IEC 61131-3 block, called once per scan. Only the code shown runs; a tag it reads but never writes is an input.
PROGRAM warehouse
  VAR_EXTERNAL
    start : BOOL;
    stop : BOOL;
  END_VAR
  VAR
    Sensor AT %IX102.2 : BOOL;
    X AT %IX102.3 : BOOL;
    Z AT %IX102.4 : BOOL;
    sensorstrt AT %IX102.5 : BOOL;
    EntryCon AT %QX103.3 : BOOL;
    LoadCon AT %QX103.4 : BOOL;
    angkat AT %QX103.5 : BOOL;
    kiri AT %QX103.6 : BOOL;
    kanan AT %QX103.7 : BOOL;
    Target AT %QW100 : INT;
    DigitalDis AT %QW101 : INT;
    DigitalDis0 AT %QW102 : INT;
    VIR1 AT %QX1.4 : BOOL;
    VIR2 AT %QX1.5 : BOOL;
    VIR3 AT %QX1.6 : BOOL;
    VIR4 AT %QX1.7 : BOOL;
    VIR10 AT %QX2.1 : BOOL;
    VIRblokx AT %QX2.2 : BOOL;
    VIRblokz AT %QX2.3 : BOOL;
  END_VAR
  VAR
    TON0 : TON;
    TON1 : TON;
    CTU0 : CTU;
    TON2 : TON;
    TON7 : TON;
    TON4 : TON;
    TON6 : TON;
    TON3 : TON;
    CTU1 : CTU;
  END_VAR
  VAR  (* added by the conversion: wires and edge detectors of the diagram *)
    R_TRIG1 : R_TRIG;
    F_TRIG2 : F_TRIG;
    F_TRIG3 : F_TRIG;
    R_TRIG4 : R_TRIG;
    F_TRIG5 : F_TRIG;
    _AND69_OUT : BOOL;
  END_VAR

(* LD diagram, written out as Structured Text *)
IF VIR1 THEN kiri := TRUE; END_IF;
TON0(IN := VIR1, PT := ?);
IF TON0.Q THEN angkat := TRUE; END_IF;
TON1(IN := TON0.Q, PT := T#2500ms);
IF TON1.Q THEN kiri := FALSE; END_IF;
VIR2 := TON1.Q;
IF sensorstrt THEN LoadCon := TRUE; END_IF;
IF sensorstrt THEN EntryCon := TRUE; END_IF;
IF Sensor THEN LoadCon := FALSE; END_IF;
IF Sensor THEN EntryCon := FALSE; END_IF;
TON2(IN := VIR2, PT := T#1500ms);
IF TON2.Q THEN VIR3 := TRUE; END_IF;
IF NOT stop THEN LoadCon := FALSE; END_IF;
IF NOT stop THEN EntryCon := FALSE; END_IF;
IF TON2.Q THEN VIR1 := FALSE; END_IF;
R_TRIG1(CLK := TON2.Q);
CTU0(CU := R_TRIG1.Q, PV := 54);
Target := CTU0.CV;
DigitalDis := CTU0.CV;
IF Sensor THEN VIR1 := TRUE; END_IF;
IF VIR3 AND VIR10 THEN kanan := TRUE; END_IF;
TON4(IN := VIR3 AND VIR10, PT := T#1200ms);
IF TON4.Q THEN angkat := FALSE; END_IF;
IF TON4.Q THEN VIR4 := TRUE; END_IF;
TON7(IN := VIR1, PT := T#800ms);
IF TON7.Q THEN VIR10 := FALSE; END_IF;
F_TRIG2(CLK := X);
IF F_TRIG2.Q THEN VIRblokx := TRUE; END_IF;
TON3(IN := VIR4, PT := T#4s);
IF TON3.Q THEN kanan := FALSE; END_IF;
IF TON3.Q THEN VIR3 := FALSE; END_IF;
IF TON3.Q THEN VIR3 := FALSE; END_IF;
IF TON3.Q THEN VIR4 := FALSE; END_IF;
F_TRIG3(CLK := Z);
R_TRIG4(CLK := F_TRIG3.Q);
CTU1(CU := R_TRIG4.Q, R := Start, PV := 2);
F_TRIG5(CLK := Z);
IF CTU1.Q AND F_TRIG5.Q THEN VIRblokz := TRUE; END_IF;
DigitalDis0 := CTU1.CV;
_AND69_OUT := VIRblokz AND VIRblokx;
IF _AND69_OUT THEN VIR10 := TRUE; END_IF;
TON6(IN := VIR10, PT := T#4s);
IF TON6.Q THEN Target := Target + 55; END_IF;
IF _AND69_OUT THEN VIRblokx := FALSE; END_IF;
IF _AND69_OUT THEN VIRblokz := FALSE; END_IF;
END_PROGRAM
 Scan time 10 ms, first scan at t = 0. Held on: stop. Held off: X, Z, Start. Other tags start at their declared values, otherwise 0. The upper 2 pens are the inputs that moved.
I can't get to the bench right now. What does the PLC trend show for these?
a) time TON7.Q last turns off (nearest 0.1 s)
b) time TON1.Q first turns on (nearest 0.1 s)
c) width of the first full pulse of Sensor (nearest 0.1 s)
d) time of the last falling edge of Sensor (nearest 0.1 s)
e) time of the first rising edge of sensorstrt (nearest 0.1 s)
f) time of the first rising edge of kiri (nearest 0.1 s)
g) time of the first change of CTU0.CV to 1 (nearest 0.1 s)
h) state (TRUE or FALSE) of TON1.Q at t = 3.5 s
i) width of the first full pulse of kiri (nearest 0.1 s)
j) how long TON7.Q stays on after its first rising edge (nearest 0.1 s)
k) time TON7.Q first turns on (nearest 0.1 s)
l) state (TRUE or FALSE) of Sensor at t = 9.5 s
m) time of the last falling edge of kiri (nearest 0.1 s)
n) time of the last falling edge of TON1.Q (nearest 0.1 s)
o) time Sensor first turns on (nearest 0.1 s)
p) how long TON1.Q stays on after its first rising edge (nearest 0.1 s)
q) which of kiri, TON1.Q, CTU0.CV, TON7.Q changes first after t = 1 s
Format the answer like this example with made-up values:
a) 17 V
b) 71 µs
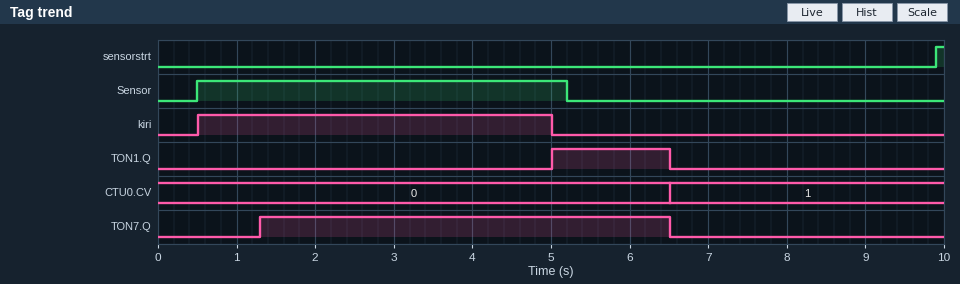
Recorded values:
a) 6.5 s
b) 5.0 s
c) 4.7 s
d) 5.2 s
e) 9.9 s
f) 0.5 s
g) 6.5 s
h) FALSE
i) 4.5 s
j) 5.2 s
k) 1.3 s
l) FALSE
m) 5.0 s
n) 6.5 s
o) 0.5 s
p) 1.5 s
q) TON7.Q
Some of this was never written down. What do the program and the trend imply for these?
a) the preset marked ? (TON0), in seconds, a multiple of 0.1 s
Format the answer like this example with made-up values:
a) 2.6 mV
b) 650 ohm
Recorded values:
a) 2.0 s
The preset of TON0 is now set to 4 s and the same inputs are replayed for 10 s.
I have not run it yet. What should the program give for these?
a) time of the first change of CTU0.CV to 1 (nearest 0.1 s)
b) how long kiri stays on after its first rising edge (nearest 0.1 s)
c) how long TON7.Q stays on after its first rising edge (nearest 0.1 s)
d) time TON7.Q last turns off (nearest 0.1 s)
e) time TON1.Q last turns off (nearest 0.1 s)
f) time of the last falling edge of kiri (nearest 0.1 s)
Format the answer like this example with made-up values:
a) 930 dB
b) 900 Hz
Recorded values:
a) 8.5 s
b) 6.5 s
c) 7.2 s
d) 8.5 s
e) 8.5 s
f) 7.0 s
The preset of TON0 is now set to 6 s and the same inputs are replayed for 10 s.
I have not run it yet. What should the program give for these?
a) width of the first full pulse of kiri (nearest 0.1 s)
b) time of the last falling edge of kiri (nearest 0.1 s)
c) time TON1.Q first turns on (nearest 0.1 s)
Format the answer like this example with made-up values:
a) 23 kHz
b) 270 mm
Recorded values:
a) 8.5 s
b) 9.0 s
c) 9.0 s
